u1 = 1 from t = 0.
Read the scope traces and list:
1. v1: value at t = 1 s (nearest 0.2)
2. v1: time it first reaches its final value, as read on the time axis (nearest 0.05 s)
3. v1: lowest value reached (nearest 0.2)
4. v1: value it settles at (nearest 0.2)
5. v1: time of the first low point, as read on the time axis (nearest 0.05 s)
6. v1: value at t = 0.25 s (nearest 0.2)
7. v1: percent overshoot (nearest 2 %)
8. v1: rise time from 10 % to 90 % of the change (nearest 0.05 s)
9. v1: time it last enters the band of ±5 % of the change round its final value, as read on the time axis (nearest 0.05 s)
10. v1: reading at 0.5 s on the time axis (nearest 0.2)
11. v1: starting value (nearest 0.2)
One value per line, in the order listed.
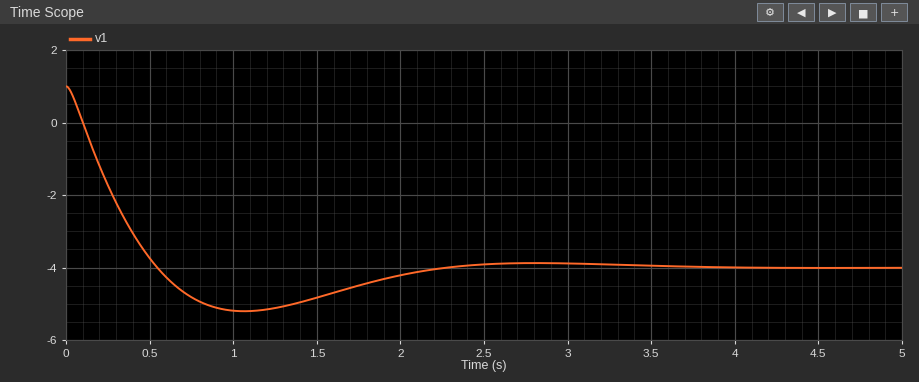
-5.2
0.55 s
-5.2
-4.0
1.05 s
-1.8
24 %
0.40 s
1.95 s
-3.8
1.0
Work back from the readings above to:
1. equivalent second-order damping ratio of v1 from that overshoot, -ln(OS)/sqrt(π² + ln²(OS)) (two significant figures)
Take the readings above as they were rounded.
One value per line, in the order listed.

0.41
